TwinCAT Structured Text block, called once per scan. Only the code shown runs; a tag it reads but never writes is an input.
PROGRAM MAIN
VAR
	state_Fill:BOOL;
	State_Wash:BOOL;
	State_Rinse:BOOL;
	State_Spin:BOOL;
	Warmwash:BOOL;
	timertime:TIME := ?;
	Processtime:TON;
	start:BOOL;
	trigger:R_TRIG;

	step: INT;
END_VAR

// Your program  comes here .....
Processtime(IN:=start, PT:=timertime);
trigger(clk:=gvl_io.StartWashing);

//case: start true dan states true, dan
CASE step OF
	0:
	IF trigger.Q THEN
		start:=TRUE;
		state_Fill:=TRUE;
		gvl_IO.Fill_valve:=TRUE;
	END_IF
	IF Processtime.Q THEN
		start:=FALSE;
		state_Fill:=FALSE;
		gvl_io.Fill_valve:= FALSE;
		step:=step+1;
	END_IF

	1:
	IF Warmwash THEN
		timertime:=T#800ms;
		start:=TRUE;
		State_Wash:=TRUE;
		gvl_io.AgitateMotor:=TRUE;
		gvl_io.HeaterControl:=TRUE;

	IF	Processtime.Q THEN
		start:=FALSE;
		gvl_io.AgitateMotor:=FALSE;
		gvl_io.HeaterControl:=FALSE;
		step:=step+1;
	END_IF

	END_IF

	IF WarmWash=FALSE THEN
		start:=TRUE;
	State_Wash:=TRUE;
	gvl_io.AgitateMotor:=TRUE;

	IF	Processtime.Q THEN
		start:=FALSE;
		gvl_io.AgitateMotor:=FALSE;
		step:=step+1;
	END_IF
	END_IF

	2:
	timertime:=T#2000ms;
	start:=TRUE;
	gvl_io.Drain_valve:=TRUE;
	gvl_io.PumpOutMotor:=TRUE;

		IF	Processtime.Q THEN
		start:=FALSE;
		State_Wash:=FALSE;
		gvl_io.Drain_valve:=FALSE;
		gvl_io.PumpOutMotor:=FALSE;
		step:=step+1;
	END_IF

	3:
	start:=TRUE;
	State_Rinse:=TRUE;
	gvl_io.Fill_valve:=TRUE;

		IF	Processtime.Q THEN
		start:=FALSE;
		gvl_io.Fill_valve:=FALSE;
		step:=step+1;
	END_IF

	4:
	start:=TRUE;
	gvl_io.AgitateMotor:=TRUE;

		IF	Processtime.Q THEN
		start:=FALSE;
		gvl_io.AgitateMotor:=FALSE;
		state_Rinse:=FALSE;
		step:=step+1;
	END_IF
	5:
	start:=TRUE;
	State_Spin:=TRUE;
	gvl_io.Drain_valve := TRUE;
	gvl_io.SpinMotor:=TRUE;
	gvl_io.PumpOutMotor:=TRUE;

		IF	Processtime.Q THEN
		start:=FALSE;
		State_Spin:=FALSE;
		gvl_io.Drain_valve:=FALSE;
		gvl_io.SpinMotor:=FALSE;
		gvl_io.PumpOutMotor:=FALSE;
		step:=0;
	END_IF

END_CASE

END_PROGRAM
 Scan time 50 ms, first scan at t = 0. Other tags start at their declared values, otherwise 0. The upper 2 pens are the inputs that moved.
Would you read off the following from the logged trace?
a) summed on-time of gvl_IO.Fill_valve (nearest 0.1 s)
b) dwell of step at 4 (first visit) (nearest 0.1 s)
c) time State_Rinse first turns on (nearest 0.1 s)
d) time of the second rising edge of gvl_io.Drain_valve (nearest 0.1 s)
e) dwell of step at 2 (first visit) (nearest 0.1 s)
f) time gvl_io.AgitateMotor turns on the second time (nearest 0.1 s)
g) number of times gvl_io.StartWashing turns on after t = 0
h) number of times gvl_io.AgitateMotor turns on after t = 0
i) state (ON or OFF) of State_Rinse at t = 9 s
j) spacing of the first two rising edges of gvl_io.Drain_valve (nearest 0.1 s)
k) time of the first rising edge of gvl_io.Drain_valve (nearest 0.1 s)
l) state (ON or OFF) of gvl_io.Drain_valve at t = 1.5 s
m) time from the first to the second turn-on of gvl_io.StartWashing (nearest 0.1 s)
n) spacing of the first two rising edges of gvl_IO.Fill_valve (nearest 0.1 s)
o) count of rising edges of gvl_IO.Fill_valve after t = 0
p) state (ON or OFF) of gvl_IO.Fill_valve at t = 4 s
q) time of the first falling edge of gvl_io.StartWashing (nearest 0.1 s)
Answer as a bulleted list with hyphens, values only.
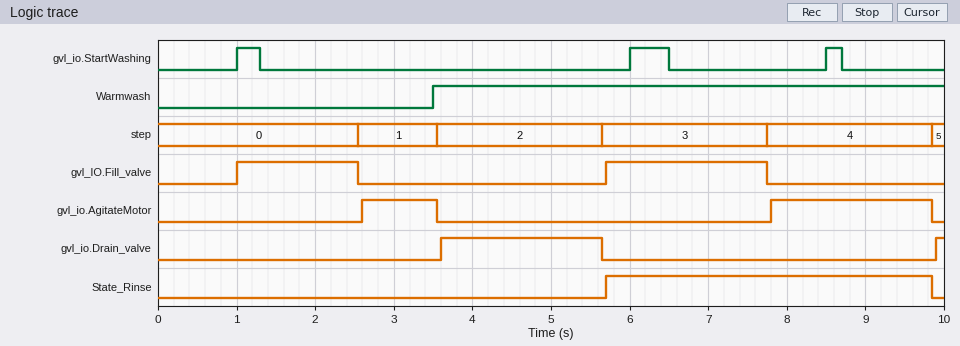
- 3.6 s
- 2.1 s
- 5.7 s
- 9.9 s
- 2.1 s
- 7.8 s
- 3
- 2
- ON
- 6.3 s
- 3.6 s
- OFF
- 5.0 s
- 4.7 s
- 2
- OFF
- 1.3 s
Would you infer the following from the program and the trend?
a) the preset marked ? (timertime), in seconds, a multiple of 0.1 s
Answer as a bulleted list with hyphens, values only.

- 1.5 s
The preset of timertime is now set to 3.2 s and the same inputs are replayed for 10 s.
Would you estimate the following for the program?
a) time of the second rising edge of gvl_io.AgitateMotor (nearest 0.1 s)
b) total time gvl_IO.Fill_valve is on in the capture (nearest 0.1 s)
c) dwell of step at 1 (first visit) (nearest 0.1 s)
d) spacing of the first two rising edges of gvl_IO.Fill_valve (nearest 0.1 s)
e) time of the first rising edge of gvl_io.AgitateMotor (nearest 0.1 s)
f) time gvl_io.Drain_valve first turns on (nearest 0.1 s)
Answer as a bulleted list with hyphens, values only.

- 9.4 s
- 5.3 s
- 0.9 s
- 6.3 s
- 4.3 s
- 5.2 s
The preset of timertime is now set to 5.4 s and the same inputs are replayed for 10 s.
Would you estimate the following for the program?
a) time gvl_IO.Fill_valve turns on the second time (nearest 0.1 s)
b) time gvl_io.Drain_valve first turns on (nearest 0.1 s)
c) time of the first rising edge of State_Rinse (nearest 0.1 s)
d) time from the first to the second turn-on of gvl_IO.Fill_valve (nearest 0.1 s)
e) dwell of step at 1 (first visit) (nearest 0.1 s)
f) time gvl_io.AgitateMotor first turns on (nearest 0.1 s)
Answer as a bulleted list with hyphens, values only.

- 9.5 s
- 7.4 s
- 9.5 s
- 8.5 s
- 0.9 s
- 6.5 s
